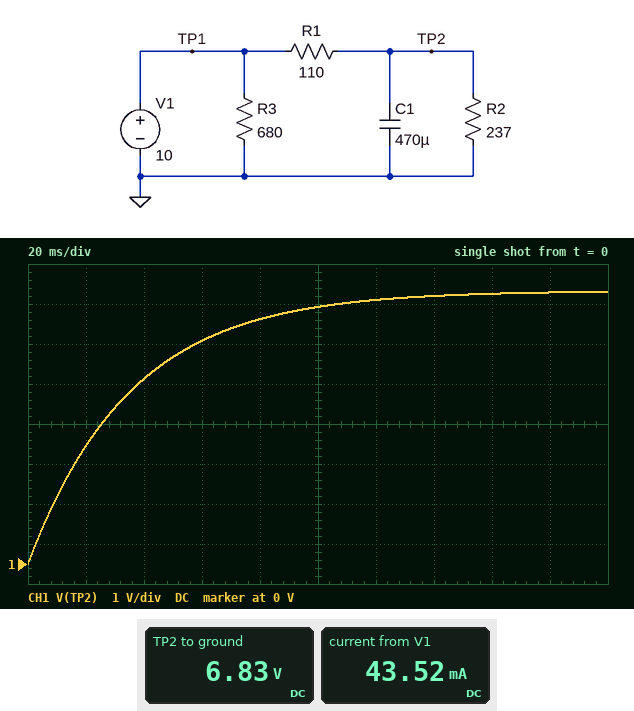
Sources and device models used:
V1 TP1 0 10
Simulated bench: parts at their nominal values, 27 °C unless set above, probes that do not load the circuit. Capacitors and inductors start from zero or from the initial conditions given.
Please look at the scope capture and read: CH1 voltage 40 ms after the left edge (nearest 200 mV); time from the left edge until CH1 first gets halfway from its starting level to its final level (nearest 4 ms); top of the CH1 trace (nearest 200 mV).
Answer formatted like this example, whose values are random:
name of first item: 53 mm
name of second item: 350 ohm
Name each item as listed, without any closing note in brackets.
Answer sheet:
CH1 voltage 40 ms after the left edge: 4.6 V
time from the left edge until CH1 first gets halfway from its starting level to its final level: 24 ms
top of the CH1 trace: 6.8 V
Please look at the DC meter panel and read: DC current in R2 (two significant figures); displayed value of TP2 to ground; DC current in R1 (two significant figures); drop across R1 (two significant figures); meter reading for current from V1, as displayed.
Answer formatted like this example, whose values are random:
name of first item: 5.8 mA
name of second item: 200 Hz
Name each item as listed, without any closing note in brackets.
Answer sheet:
DC current in R2: 29 mA
displayed value of TP2 to ground: 6.83 V
DC current in R1: 29 mA
drop across R1: 3.2 V
meter reading for current from V1, as displayed: 43.52 mA
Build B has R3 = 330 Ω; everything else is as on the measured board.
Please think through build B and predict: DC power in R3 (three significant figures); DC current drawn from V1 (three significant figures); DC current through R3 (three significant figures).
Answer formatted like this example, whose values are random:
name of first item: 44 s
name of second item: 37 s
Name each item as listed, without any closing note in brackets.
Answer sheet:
DC power in R3: 303 mW
DC current drawn from V1: 59.1 mA
DC current through R3: 30.3 mA
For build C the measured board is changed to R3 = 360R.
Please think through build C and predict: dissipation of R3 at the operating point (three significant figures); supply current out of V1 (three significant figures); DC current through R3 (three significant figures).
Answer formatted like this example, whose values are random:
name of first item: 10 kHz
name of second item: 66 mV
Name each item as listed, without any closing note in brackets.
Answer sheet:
dissipation of R3 at the operating point: 278 mW
supply current out of V1: 56.6 mA
DC current through R3: 27.8 mA
